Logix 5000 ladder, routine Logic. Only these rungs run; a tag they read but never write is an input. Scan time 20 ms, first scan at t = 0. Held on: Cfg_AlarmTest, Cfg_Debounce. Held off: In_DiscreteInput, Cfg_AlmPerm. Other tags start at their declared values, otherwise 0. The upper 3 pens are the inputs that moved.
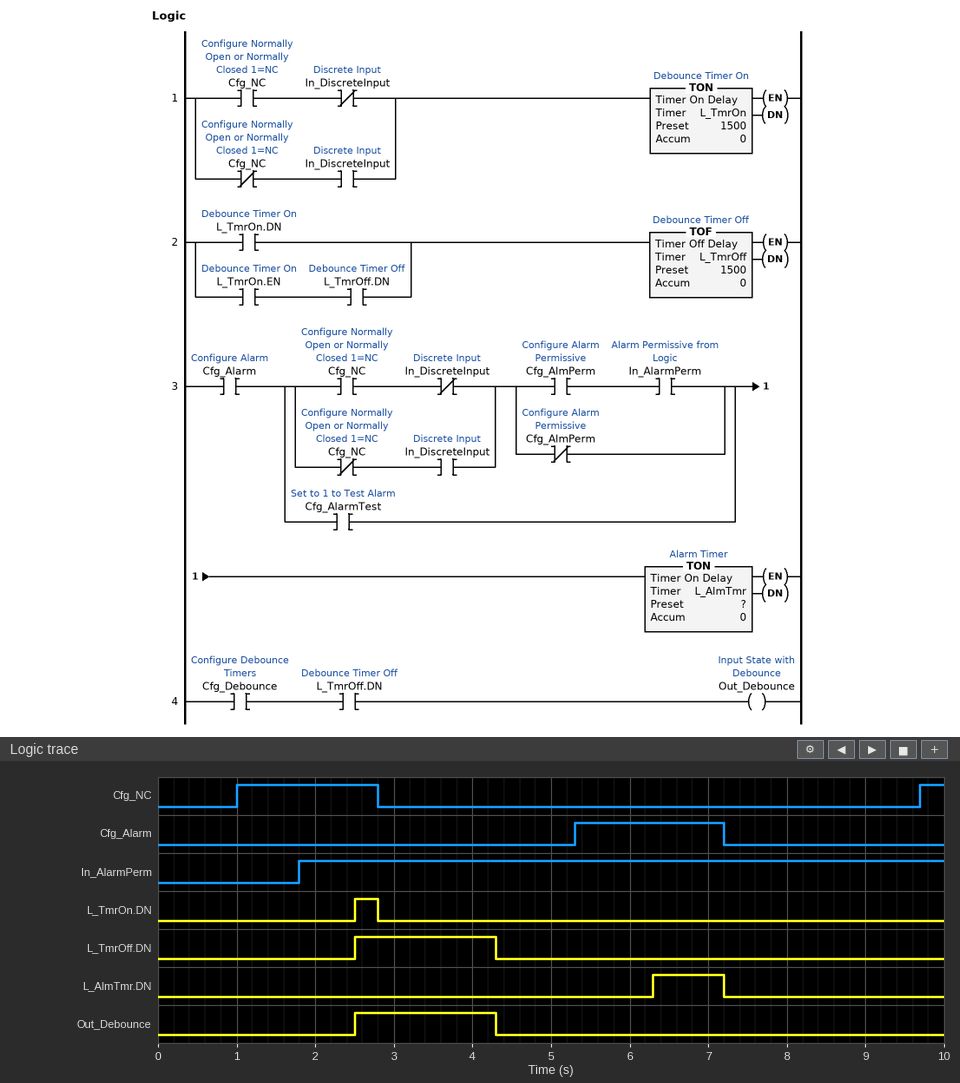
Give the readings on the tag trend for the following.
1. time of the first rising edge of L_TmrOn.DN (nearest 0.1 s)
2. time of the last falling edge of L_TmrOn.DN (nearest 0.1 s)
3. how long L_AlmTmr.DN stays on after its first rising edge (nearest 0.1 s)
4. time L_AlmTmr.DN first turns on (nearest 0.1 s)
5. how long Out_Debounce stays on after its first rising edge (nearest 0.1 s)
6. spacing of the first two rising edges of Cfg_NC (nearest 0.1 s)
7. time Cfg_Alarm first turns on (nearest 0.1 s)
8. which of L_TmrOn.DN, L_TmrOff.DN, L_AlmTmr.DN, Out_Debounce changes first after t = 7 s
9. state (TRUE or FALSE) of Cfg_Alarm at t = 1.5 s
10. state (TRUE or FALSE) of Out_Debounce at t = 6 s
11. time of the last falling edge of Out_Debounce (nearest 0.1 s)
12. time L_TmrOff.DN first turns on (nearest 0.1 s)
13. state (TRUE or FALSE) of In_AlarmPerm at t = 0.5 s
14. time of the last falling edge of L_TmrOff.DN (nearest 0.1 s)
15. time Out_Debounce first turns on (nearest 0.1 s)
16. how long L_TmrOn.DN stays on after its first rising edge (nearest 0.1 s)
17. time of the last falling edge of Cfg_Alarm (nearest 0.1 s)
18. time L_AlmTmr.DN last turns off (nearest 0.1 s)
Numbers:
2.5 s
2.8 s
0.9 s
6.3 s
1.8 s
8.7 s
5.3 s
L_AlmTmr.DN
FALSE
FALSE
4.3 s
2.5 s
FALSE
4.3 s
2.5 s
0.3 s
7.2 s
7.2 s
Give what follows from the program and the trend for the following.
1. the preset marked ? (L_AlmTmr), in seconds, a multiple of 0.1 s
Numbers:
1.0 s
